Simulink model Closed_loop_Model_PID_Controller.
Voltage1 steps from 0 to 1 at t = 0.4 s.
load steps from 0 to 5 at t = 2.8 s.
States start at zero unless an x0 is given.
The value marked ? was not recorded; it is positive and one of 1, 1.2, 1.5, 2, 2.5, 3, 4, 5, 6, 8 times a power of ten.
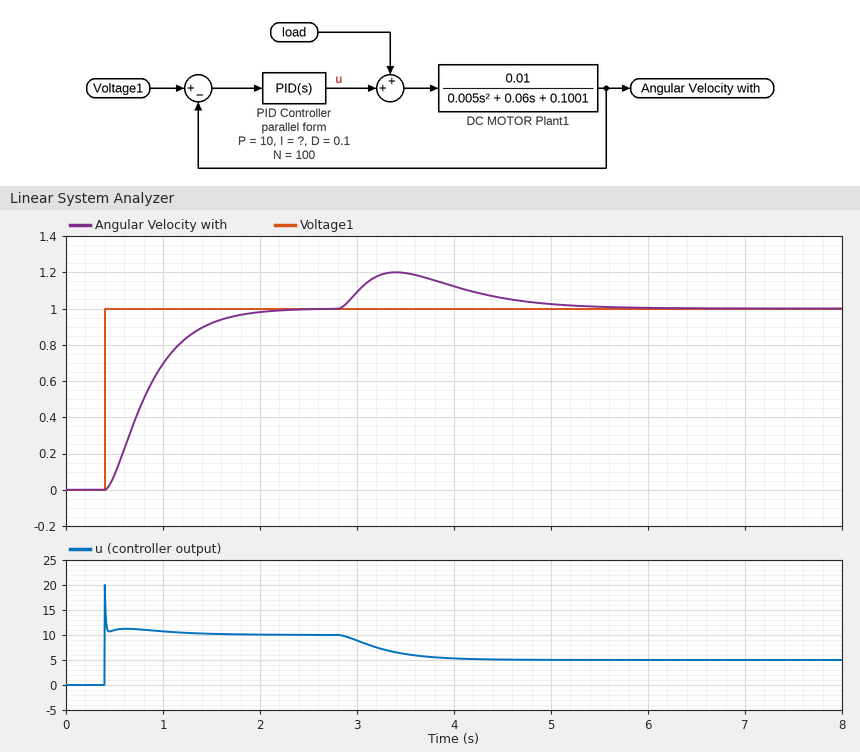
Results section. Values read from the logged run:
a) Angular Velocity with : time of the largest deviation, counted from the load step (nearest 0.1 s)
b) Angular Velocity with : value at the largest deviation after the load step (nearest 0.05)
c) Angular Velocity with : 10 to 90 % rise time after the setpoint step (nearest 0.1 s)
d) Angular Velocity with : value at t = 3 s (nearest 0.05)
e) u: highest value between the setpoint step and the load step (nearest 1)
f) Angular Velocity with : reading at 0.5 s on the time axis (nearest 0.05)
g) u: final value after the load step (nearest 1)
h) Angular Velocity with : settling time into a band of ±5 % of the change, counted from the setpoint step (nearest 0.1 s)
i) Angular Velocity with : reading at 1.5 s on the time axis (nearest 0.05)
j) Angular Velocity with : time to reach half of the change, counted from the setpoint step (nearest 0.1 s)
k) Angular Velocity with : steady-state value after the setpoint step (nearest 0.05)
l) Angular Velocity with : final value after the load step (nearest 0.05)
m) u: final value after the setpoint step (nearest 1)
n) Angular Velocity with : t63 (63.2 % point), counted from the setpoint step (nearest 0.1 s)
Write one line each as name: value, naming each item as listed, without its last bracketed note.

Angular Velocity with : time of the largest deviation, counted from the load step: 0.6 s
Angular Velocity with : value at the largest deviation after the load step: 1.20
Angular Velocity with : 10 to 90 % rise time after the setpoint step: 0.9 s
Angular Velocity with : value at t = 3 s: 1.10
u: highest value between the setpoint step and the load step: 20
Angular Velocity with : reading at 0.5 s on the time axis: 0.10
u: final value after the load step: 5
Angular Velocity with : settling time into a band of ±5 % of the change, counted from the setpoint step: 1.3 s
Angular Velocity with : reading at 1.5 s on the time axis: 0.90
Angular Velocity with : time to reach half of the change, counted from the setpoint step: 0.4 s
Angular Velocity with : steady-state value after the setpoint step: 1.00
Angular Velocity with : final value after the load step: 1.00
u: final value after the setpoint step: 10
Angular Velocity with : t63 (63.2 % point), counted from the setpoint step: 0.5 s
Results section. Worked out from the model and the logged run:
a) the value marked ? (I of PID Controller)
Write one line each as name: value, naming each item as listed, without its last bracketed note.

the value marked ?: 20
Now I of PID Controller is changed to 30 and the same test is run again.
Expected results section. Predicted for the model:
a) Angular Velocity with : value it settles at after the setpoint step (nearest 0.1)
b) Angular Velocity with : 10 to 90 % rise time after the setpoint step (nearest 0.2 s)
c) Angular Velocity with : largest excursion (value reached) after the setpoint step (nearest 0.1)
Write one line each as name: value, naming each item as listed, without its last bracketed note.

Angular Velocity with : value it settles at after the setpoint step: 1.0
Angular Velocity with : 10 to 90 % rise time after the setpoint step: 0.6 s
Angular Velocity with : largest excursion (value reached) after the setpoint step: 1.1
